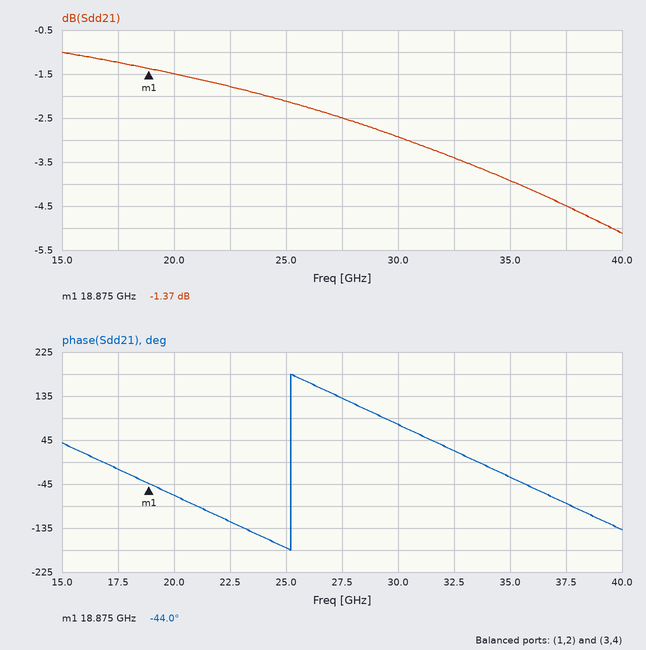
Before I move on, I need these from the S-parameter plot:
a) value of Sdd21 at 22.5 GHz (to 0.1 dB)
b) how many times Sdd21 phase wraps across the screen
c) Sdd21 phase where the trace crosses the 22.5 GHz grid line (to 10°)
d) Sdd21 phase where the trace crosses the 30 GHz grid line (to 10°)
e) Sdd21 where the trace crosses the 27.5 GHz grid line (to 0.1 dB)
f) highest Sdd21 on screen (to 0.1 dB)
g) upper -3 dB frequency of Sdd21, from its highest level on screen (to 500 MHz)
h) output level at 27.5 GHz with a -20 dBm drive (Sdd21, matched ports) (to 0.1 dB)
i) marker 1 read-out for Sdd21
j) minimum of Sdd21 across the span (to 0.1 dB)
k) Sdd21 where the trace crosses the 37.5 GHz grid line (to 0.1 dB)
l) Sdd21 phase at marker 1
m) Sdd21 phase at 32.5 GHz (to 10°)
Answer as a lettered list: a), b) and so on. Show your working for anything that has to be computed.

a) -1.8 dB
b) 1
c) -120°
d) 80°
e) -2.5 dB
f) -1.0 dB
g) 35.5 GHz
h) -20 dBm + (-2.5 dB) = -22.5 dBm
i) -1.37 dB
j) -5.1 dB
k) -4.5 dB
l) -44.0°
m) 20°
